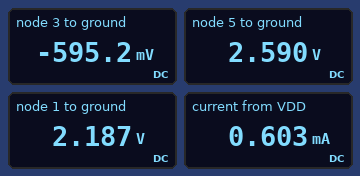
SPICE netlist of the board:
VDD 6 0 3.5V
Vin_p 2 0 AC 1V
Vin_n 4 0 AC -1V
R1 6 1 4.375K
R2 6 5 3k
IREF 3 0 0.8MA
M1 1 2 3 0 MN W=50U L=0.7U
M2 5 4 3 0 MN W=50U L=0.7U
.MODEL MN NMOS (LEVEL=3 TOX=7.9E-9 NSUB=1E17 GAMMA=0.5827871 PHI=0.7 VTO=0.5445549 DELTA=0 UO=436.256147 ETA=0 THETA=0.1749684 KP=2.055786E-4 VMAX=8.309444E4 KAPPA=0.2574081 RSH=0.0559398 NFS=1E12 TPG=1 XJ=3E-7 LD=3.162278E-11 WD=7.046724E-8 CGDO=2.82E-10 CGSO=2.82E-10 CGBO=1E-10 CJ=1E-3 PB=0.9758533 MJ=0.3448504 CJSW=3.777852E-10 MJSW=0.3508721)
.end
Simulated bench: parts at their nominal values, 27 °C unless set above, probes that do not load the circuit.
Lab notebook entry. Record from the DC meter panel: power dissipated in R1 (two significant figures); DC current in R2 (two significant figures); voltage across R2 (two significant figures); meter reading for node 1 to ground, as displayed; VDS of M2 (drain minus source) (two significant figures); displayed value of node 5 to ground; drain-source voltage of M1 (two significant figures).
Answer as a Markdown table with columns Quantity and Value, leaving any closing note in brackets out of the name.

| Quantity | Value |
|---|---|
| power dissipated in R1 | 390 µW |
| DC current in R2 | 300 µA |
| voltage across R2 | 910 mV |
| meter reading for node 1 to ground, as displayed | 2.187 V |
| VDS of M2 (drain minus source) | 3.2 V |
| displayed value of node 5 to ground | 2.590 V |
| drain-source voltage of M1 | 2.8 V |
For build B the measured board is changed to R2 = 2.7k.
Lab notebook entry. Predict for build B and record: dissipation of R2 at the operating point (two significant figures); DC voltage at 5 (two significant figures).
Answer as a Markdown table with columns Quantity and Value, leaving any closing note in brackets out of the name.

| Quantity | Value |
|---|---|
| dissipation of R2 at the operating point | 250 µW |
| DC voltage at 5 | 2.7 V |
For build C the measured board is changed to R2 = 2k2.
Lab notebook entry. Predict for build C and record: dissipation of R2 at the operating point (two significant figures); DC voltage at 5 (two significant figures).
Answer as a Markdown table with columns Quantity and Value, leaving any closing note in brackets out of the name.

| Quantity | Value |
|---|---|
| dissipation of R2 at the operating point | 200 µW |
| DC voltage at 5 | 2.8 V |
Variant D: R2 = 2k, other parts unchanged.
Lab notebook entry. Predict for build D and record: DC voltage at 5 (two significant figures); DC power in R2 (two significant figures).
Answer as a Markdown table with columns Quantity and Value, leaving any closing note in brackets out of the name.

| Quantity | Value |
|---|---|
| DC voltage at 5 | 2.9 V |
| DC power in R2 | 190 µW |
